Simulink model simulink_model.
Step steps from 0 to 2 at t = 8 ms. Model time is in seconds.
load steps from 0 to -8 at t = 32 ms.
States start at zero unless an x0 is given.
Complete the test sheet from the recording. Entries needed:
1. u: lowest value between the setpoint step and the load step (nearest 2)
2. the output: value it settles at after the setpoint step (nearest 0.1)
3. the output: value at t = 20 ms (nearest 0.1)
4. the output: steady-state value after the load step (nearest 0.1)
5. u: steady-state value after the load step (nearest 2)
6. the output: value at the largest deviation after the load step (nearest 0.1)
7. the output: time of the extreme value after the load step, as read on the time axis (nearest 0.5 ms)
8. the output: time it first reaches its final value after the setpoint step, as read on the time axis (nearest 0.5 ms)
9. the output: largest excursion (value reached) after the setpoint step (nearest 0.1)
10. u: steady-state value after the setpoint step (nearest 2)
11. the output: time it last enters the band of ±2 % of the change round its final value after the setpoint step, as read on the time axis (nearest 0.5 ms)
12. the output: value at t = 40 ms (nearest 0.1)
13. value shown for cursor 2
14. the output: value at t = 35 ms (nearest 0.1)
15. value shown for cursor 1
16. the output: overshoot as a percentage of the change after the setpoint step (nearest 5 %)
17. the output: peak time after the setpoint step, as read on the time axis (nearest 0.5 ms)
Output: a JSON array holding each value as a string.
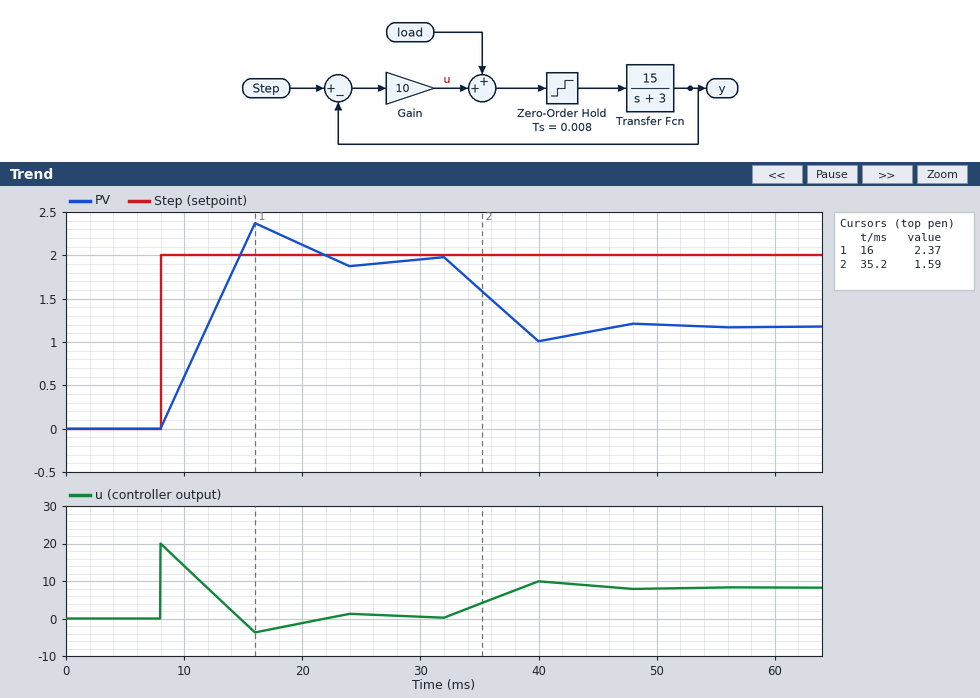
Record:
["-4", "2.0", "2.1", "1.2", "8", "1.0", "40.0 ms", "14.5 ms", "2.4", "0", "27.5 ms", "1.0", "1.59", "1.6", "2.37", "20 %", "16.0 ms"]
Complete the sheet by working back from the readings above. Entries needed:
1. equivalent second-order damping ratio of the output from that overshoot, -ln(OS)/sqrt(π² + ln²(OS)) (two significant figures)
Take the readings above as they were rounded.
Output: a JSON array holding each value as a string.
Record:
["0.46"]
